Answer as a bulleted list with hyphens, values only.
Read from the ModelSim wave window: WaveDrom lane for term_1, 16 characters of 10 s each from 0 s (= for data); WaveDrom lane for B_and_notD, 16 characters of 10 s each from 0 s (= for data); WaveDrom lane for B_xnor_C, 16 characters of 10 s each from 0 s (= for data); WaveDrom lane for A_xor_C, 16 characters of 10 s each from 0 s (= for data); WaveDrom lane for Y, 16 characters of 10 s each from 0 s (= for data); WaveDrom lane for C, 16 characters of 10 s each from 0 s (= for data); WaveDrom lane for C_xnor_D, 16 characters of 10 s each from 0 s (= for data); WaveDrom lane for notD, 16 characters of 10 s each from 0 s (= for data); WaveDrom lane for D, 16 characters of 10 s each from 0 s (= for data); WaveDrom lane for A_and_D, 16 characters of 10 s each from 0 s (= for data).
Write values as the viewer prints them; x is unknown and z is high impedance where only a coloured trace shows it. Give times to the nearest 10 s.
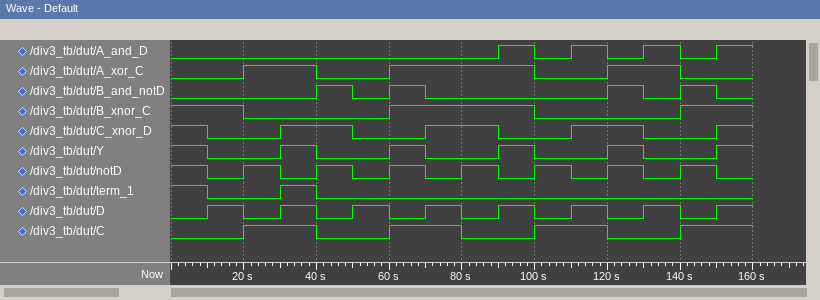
- {name: 'term_1', wave: '10.10...........'}
- {name: 'B_and_notD', wave: '0...1010....1010'}
- {name: 'B_xnor_C', wave: '1.0...1...0...1.'}
- {name: 'A_xor_C', wave: '0.1.0.1...0.1.0.'}
- {name: 'Y', wave: '10.10.10.10.10.1'}
- {name: 'C', wave: '0.1.0.1.0.1.0.1.'}
- {name: 'C_xnor_D', wave: '10.1.0.1.0.1.0.1'}
- {name: 'notD', wave: '1010101010101010'}
- {name: 'D', wave: '0101010101010101'}
- {name: 'A_and_D', wave: '0........1010101'}
